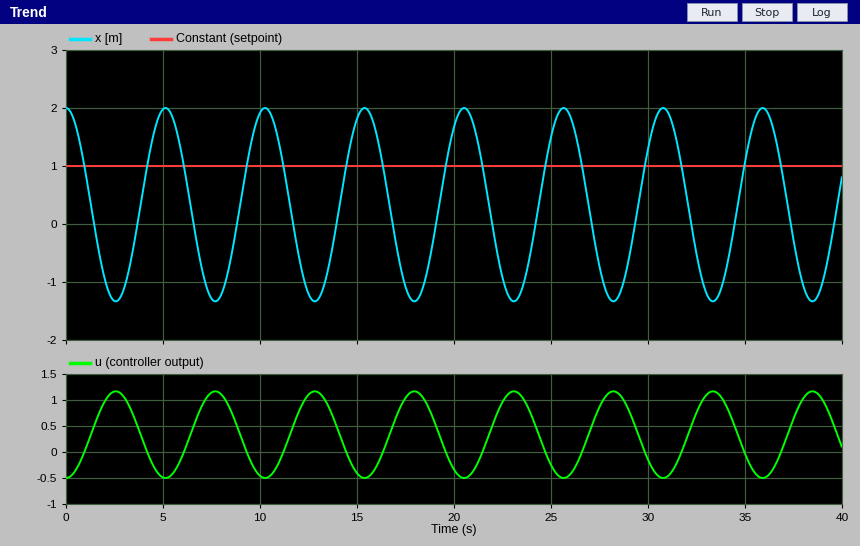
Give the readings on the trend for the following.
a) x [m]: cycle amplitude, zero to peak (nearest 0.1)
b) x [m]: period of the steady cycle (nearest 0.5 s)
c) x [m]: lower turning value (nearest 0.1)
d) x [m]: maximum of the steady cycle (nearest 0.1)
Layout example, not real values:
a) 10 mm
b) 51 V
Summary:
a) 1.7
b) 5.0 s
c) -1.3
d) 2.0
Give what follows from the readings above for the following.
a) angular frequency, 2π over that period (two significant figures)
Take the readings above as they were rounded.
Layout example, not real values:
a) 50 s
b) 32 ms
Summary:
a) 1.3 rad/s
